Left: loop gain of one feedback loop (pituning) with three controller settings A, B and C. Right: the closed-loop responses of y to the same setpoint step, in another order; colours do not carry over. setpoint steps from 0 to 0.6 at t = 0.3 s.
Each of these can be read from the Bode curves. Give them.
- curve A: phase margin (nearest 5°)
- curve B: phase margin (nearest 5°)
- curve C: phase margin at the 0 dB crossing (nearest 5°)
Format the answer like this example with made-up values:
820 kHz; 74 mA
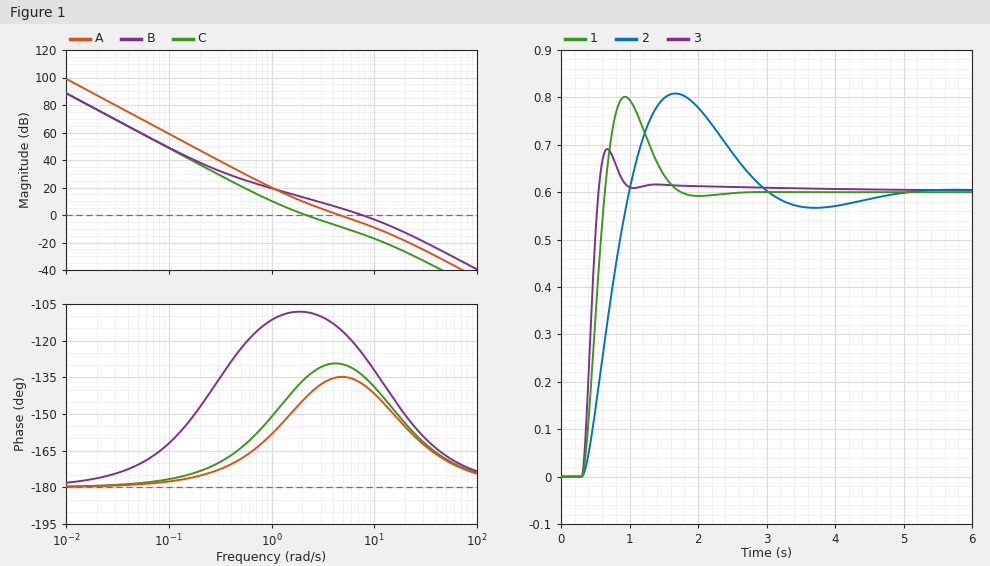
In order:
45°; 55°; 45°
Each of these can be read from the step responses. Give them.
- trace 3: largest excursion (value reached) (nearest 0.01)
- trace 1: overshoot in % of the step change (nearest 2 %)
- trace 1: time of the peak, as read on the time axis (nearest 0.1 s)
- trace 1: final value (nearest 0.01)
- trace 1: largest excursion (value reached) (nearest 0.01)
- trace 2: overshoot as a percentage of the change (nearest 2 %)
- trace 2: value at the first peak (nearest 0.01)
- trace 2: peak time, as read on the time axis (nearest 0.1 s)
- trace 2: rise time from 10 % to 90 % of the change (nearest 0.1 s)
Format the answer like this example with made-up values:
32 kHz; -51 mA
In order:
0.69; 34 %; 0.9 s; 0.60; 0.80; 34 %; 0.81; 1.7 s; 0.5 s
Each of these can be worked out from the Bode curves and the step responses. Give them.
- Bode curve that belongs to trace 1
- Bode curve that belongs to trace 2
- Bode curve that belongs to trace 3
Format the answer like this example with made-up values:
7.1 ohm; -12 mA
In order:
A; C; B
